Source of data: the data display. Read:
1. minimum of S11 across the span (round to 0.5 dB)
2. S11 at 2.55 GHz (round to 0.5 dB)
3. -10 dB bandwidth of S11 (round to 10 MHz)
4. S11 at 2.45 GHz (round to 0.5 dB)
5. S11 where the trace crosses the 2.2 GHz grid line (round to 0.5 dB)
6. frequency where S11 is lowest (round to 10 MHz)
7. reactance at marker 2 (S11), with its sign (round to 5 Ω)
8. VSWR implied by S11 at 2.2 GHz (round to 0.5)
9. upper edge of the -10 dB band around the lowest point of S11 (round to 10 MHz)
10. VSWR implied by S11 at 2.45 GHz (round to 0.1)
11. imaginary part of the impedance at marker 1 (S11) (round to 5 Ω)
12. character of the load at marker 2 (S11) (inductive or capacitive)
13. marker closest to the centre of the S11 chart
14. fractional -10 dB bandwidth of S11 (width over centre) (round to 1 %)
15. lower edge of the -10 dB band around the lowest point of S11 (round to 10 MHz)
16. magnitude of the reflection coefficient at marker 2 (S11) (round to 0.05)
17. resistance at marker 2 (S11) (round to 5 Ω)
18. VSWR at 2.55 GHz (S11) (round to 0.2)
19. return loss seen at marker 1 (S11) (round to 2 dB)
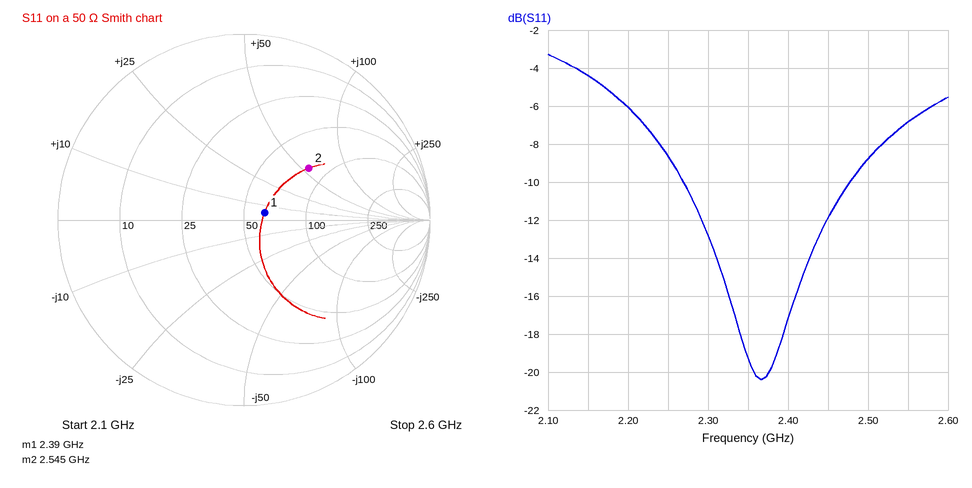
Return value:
-20.5 dB
-7.0 dB
210 MHz
-12.0 dB
-6.0 dB
2.37 GHz
+55 Ω
3.0
2.48 GHz
1.7
+5 Ω
inductive
marker 1
9 %
2.27 GHz
0.45
80 Ω
2.6
18 dB
